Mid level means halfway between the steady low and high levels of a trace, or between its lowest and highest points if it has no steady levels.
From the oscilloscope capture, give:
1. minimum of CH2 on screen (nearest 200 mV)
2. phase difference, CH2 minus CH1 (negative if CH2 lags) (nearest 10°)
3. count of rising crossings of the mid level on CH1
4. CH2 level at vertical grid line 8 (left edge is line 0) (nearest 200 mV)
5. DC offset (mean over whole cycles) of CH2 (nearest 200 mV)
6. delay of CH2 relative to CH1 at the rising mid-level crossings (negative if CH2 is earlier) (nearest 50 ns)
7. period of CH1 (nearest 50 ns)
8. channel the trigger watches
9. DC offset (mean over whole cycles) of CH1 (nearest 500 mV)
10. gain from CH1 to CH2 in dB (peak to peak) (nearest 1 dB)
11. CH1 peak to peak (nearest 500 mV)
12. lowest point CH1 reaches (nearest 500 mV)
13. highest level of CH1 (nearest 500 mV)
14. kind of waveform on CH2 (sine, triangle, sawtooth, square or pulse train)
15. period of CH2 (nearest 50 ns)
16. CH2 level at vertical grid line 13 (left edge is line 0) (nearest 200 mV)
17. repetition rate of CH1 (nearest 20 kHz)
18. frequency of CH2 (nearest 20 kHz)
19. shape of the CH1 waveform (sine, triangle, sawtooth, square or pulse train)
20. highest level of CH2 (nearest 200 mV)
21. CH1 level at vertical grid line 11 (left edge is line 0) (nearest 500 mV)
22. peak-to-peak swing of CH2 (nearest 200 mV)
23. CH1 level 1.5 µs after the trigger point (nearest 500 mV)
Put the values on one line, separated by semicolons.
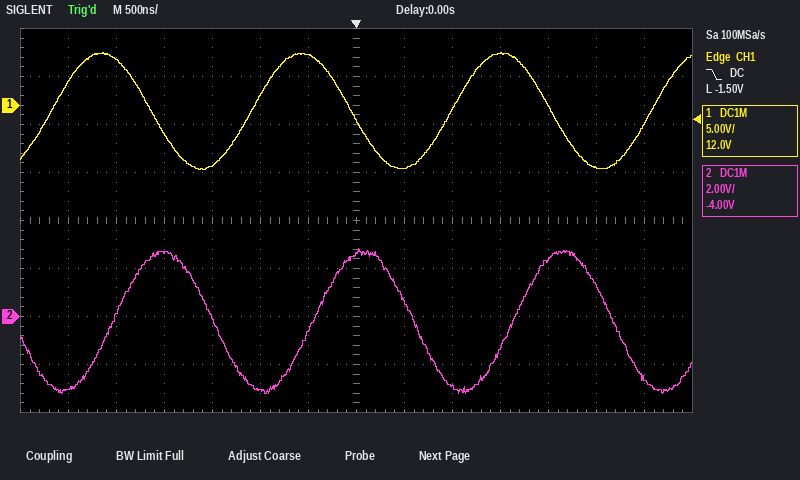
-3.2 V; -110°; 4; 600 mV; -200 mV; +650 ns; 2.10 µs; CH1; -500 mV; -6 dB; 12.0 V; -6.5 V; 5.5 V; sine; 2.10 µs; -2.6 V; 480 kHz; 480 kHz; sine; 2.8 V; 0.0 V; 6.0 V; 5.5 V
